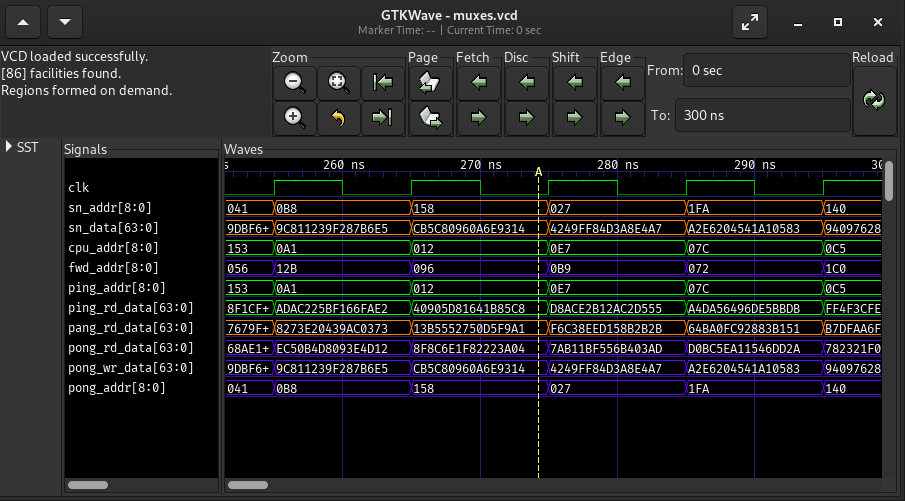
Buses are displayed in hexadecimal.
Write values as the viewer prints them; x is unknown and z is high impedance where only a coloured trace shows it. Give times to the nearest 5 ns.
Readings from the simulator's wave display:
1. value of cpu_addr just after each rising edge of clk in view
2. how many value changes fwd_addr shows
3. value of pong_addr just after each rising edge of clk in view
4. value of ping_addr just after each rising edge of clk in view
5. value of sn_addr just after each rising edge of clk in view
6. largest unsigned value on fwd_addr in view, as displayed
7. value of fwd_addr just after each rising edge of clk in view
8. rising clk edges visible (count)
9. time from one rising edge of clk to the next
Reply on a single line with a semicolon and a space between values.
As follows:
0A1, 012, 0E7, 07C, 0C5; 5; 0B8, 158, 027, 1FA, 140; 0A1, 012, 0E7, 07C, 0C5; 0B8, 158, 027, 1FA, 140; 1C0; 12B, 096, 0B9, 072, 1C0; 5; 10 ns
